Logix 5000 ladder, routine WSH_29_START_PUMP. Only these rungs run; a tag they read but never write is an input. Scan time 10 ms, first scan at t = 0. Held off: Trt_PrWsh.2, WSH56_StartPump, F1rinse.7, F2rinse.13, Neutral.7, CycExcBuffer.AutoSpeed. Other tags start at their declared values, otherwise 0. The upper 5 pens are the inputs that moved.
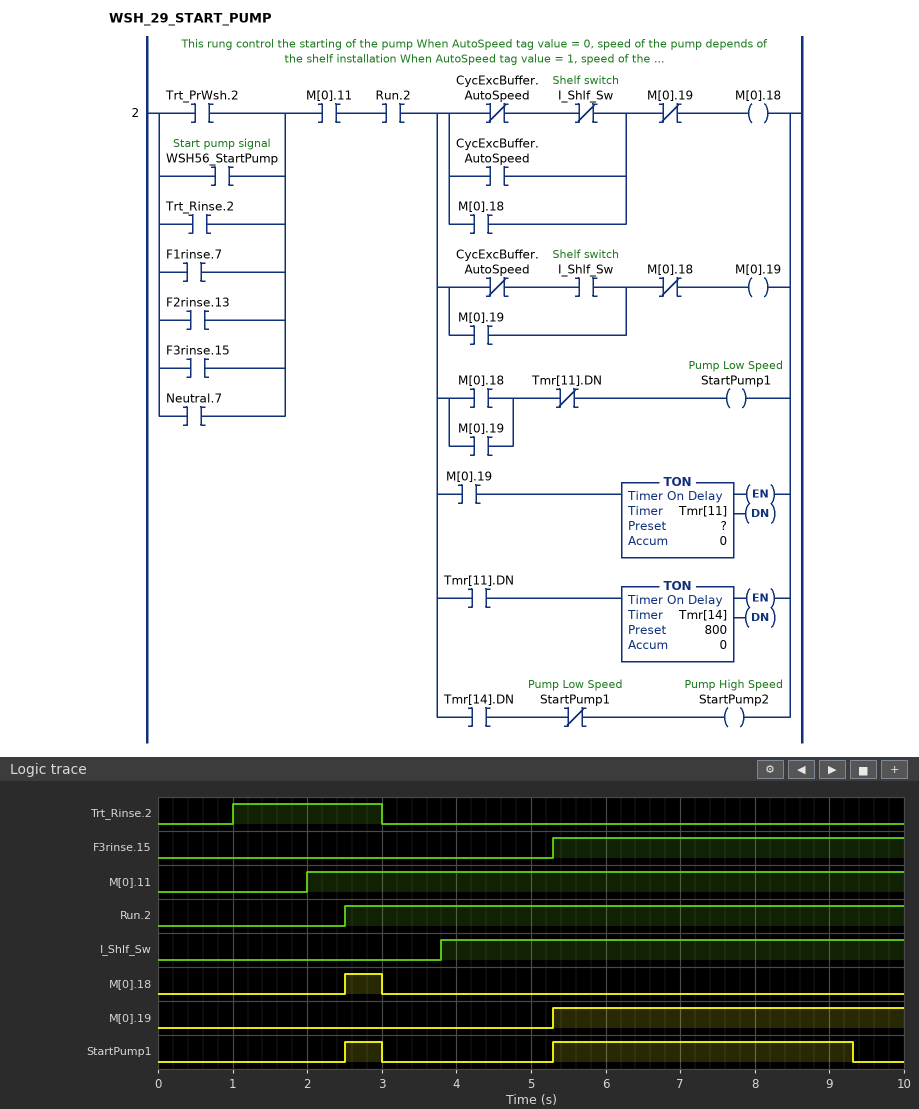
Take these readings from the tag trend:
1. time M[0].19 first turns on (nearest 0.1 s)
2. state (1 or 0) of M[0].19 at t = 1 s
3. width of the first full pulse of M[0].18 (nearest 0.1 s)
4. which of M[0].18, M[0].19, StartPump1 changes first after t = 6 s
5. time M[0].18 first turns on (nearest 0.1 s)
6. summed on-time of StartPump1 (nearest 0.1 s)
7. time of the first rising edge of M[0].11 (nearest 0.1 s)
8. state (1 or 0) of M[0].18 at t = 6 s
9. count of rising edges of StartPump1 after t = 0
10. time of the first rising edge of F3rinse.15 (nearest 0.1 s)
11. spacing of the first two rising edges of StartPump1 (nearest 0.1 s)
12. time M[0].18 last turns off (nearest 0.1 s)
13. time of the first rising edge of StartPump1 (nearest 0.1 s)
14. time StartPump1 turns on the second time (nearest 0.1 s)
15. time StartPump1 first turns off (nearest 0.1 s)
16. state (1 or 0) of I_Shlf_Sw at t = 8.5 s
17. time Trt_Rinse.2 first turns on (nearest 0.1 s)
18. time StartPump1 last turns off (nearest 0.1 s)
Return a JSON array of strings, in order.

["5.3 s", "0", "0.5 s", "StartPump1", "2.5 s", "4.5 s", "2.0 s", "0", "2", "5.3 s", "2.8 s", "3.0 s", "2.5 s", "5.3 s", "3.0 s", "1", "1.0 s", "9.3 s"]
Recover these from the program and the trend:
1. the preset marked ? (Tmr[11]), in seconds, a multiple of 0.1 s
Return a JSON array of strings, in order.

["4.0 s"]
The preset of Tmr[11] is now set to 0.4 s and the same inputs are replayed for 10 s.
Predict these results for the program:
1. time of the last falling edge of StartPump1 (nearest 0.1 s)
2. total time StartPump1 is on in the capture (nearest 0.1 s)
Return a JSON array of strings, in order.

["5.7 s", "0.9 s"]
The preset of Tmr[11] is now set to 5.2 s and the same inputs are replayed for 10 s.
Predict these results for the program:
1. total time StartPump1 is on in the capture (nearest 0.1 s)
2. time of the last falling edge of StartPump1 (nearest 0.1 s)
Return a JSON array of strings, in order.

["5.2 s", "3.0 s"]
